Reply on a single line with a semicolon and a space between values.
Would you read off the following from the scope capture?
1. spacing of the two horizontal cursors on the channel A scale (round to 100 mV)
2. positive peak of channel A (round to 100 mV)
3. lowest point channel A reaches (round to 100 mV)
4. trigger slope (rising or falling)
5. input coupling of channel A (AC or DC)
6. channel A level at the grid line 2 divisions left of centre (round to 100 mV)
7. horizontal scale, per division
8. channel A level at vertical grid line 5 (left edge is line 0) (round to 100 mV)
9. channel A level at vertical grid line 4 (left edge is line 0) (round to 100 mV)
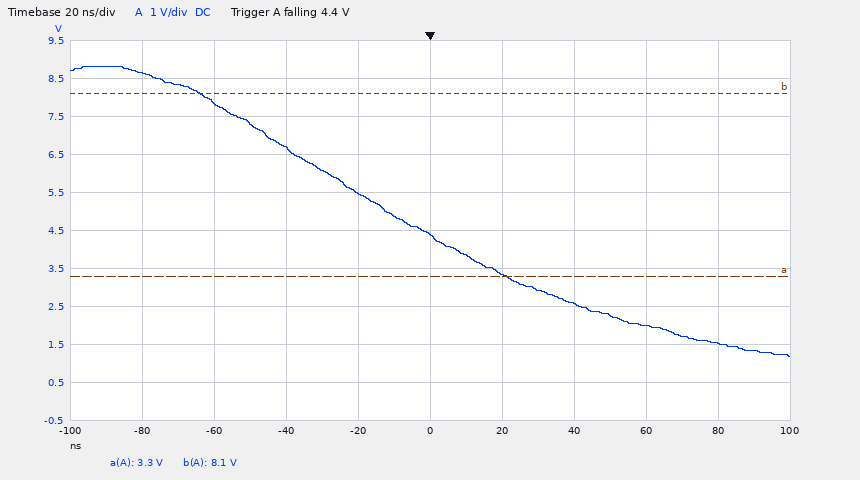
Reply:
4.8 V; 8.8 V; 1.2 V; falling; DC; 6.7 V; 20 ns; 4.4 V; 5.5 V
